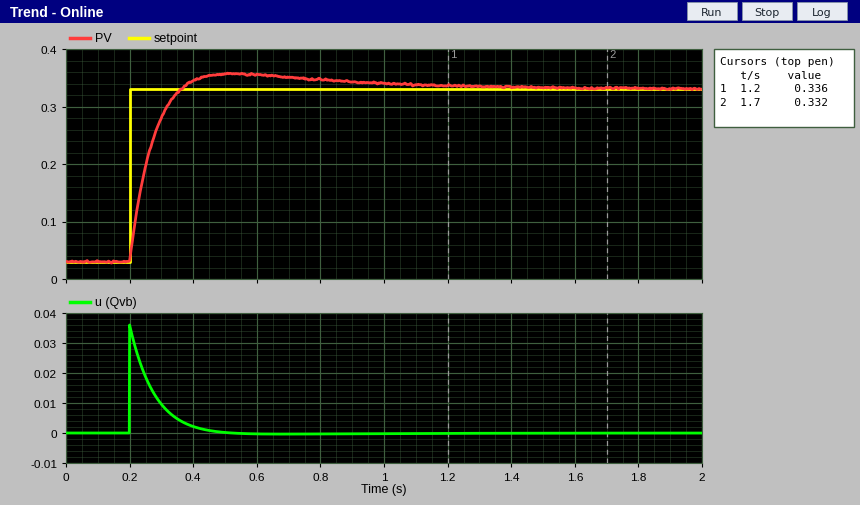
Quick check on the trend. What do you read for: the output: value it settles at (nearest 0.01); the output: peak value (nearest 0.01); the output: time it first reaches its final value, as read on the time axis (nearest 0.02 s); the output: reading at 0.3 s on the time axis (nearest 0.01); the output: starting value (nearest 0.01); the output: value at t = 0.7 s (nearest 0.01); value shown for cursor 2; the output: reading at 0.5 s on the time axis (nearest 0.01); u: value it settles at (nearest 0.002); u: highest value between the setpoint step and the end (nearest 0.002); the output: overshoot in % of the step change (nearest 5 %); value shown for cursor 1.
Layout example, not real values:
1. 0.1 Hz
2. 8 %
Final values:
1. 0.33
2. 0.36
3. 0.36 s
4. 0.28
5. 0.03
6. 0.35
7. 0.332
8. 0.36
9. 0.000
10. 0.036
11. 10 %
12. 0.336
